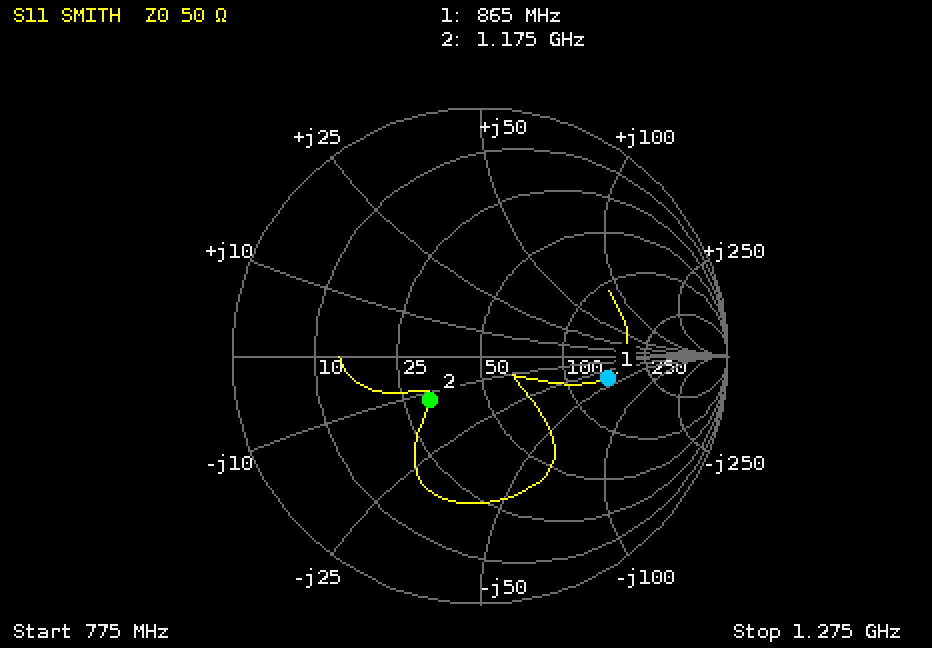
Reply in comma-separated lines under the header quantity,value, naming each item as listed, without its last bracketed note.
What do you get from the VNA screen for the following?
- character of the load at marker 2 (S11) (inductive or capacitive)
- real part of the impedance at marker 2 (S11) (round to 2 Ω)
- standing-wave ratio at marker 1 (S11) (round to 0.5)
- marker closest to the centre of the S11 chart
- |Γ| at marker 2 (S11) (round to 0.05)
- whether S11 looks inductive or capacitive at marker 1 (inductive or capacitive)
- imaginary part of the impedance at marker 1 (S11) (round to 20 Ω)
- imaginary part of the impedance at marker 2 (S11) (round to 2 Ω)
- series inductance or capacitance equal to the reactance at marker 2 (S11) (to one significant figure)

quantity,value
character of the load at marker 2 (S11),capacitive
real part of the impedance at marker 2 (S11),32 Ω
standing-wave ratio at marker 1 (S11),3.0
marker closest to the centre of the S11 chart,marker 2
|Γ| at marker 2 (S11),0.25
whether S11 looks inductive or capacitive at marker 1,capacitive
imaginary part of the impedance at marker 1 (S11),-40 Ω
imaginary part of the impedance at marker 2 (S11),-12 Ω
series inductance or capacitance equal to the reactance at marker 2 (S11),10 pF
